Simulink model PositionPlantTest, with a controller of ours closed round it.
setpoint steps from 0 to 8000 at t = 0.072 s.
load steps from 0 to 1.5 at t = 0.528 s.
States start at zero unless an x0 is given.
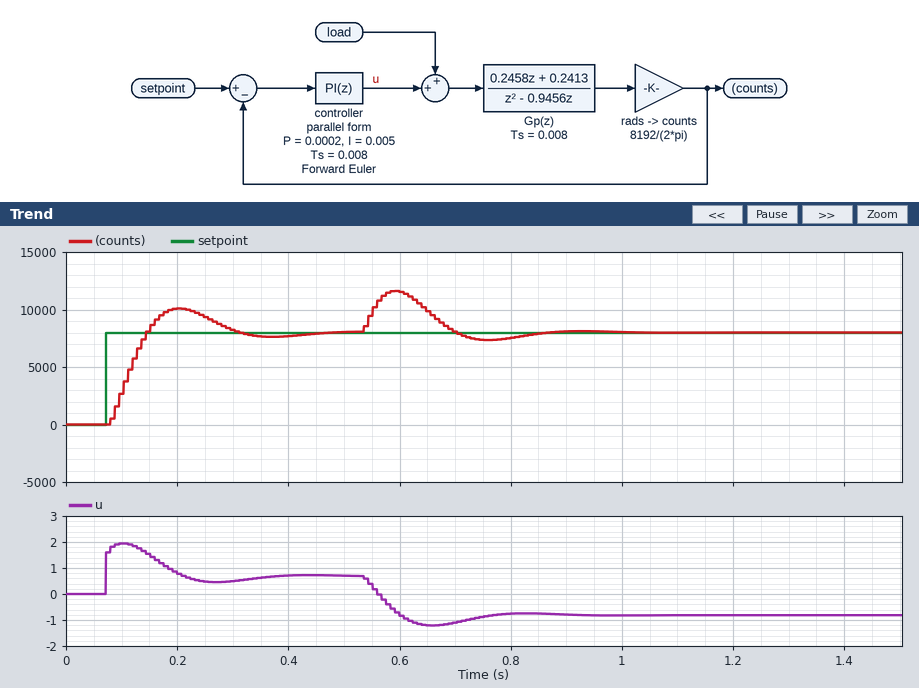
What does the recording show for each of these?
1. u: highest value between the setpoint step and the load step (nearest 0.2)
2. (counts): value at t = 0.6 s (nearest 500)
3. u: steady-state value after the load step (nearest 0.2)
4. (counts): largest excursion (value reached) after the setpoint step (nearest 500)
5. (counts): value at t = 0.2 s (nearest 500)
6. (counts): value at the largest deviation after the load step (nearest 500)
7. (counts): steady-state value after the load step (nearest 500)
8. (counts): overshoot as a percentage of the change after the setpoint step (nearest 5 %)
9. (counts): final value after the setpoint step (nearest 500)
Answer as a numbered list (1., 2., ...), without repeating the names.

1. 2.0
2. 11500
3. -0.8
4. 10000
5. 10000
6. 11500
7. 8000
8. 25 %
9. 8000
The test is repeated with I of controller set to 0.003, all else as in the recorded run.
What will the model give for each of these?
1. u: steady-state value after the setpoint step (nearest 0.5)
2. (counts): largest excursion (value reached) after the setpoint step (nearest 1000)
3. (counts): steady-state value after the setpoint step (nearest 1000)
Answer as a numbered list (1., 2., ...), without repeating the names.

1. 0.5
2. 9000
3. 8000
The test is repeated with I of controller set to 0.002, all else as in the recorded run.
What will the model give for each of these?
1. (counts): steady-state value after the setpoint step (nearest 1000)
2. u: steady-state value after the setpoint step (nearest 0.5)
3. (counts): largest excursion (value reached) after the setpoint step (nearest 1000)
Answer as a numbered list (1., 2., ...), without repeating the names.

1. 8000
2. 0.5
3. 8000
